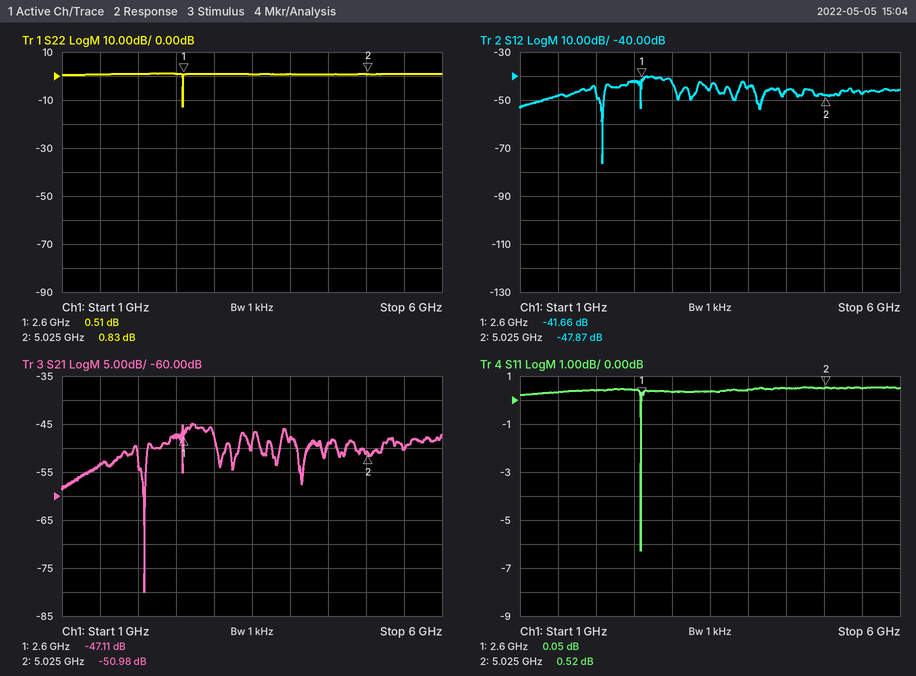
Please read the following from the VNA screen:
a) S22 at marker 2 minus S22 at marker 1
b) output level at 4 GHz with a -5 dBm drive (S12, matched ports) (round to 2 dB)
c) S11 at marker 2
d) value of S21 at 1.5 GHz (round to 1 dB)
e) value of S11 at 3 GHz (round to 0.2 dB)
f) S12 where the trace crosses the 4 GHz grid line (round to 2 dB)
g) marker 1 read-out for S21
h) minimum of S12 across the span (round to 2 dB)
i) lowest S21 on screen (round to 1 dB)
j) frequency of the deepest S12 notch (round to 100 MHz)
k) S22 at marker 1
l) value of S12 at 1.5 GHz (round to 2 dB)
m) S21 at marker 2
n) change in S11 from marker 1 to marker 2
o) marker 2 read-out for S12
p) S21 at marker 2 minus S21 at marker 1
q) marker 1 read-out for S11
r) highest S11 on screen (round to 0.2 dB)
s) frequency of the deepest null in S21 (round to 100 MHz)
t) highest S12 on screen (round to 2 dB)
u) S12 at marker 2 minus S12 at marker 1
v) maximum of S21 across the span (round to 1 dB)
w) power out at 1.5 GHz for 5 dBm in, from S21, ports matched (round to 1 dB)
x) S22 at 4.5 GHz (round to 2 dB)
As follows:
0.32 dB
-50 dBm
0.52 dB
-53 dB
0.4 dB
-44 dB
-47.11 dB
-76 dB
-80 dB
2.1 GHz
0.51 dB
-48 dB
-50.98 dB
0.47 dB
-47.87 dB
-3.87 dB
0.05 dB
0.6 dB
2.1 GHz
-40 dB
-6.21 dB
-45 dB
-48 dBm
0 dB
